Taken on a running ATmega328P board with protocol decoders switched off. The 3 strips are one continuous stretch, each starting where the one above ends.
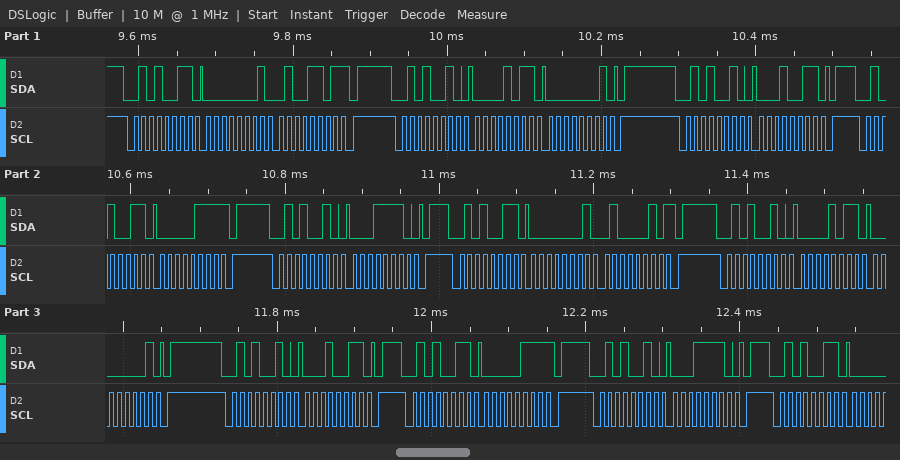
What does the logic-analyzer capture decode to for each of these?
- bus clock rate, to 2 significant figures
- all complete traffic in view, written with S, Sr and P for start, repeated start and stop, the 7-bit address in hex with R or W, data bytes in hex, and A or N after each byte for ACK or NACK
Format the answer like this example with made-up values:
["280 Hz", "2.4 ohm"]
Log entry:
["100 kHz", "S 29R A 01 A 4D N P S 29W A 0B A 01 A P S 29W A 13 A P S 29R A 07 N P S 29W A 1E A P S 29R A 01 A 42 N P S 29W A 0B A 01 A P S 29W A 13 A P S 29R A 07 N P S 29W A 1E A P S 29R A"]
